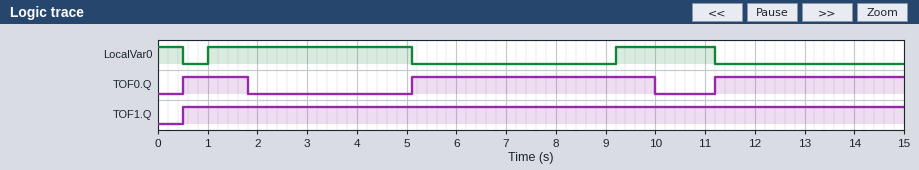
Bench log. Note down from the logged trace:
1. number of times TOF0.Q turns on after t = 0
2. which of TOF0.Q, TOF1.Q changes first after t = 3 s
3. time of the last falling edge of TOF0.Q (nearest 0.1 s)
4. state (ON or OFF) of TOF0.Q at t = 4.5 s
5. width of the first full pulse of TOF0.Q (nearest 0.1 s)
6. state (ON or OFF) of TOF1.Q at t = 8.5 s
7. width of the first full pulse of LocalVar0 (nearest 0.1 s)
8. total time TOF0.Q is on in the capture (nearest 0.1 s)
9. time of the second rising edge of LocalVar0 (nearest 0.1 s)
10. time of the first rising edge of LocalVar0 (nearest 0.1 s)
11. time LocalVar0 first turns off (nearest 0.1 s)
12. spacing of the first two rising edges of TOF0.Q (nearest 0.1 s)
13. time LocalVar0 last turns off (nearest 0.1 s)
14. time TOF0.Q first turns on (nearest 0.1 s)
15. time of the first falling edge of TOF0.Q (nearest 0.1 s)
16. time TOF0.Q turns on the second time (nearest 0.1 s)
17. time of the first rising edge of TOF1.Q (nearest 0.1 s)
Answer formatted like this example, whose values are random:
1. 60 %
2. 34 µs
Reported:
1. 3
2. TOF0.Q
3. 10.0 s
4. OFF
5. 1.3 s
6. ON
7. 4.1 s
8. 10.0 s
9. 9.2 s
10. 1.0 s
11. 0.5 s
12. 4.6 s
13. 11.2 s
14. 0.5 s
15. 1.8 s
16. 5.1 s
17. 0.5 s
